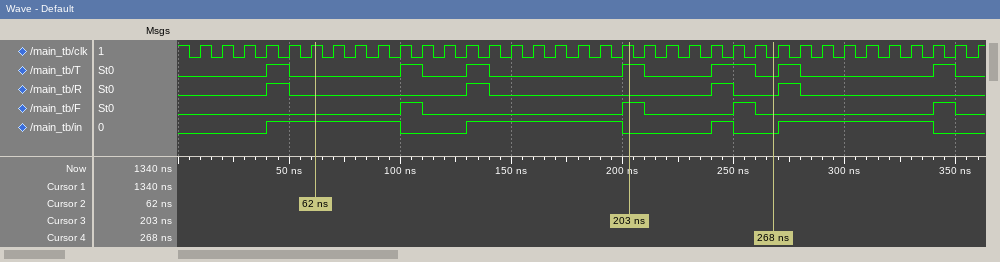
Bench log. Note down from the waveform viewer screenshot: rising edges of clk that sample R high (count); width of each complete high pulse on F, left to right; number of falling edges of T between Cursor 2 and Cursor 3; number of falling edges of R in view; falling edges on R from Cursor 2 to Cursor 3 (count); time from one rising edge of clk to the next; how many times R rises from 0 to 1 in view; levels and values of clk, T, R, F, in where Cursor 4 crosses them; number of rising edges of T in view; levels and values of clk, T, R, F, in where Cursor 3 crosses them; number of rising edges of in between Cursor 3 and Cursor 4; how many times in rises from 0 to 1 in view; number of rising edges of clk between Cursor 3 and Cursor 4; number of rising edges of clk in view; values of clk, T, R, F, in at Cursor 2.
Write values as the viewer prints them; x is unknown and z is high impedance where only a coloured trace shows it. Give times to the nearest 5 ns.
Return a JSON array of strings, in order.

["4", "10 ns, 10 ns, 10 ns, 10 ns", "2", "4", "1", "10 ns", "4", "clk=0, T=0, R=0, F=0, in=0", "7", "clk=1, T=1, R=0, F=1, in=0", "1", "4", "6", "36", "clk=1, T=0, R=0, F=0, in=1"]
